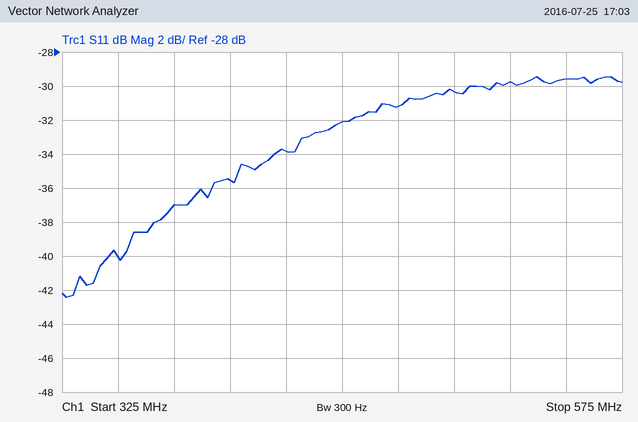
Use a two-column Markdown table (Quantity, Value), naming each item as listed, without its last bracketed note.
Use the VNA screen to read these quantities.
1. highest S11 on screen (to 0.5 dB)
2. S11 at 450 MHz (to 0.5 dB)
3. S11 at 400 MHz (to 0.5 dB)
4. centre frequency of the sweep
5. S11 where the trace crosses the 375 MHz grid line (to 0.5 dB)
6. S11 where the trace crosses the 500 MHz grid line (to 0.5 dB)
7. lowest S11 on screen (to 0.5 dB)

| Quantity | Value |
|---|---|
| highest S11 on screen | -29.5 dB |
| S11 at 450 MHz | -32.0 dB |
| S11 at 400 MHz | -35.5 dB |
| centre frequency of the sweep | 450 MHz |
| S11 where the trace crosses the 375 MHz grid line | -37.0 dB |
| S11 where the trace crosses the 500 MHz grid line | -30.5 dB |
| lowest S11 on screen | -42.5 dB |
